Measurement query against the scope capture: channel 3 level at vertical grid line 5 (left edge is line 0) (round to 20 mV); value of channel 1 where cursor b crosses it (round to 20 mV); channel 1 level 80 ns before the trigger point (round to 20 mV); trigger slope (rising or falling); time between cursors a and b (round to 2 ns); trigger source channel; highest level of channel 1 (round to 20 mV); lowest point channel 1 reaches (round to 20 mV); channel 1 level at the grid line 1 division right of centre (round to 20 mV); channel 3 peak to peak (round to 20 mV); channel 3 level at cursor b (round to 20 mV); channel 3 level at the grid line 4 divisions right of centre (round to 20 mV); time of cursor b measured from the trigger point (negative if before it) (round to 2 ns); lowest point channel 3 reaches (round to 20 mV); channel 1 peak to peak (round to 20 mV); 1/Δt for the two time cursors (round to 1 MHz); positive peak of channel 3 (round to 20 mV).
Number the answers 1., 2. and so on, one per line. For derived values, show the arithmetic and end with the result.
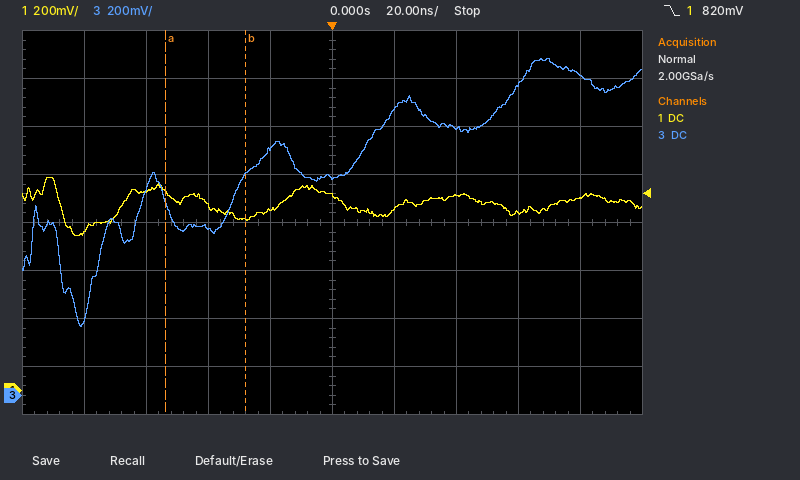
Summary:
1. 900 mV
2. 720 mV
3. 660 mV
4. falling
5. 26 ns
6. channel 1
7. 880 mV
8. 640 mV
9. 760 mV
10. 1.40 V − (280 mV) = 1.12 V
11. 920 mV
12. 1.34 V
13. -28 ns
14. 280 mV
15. 880 mV − (640 mV) = 240 mV
16. 1 / 26 ns ≈ 38 MHz
17. 1.40 V
